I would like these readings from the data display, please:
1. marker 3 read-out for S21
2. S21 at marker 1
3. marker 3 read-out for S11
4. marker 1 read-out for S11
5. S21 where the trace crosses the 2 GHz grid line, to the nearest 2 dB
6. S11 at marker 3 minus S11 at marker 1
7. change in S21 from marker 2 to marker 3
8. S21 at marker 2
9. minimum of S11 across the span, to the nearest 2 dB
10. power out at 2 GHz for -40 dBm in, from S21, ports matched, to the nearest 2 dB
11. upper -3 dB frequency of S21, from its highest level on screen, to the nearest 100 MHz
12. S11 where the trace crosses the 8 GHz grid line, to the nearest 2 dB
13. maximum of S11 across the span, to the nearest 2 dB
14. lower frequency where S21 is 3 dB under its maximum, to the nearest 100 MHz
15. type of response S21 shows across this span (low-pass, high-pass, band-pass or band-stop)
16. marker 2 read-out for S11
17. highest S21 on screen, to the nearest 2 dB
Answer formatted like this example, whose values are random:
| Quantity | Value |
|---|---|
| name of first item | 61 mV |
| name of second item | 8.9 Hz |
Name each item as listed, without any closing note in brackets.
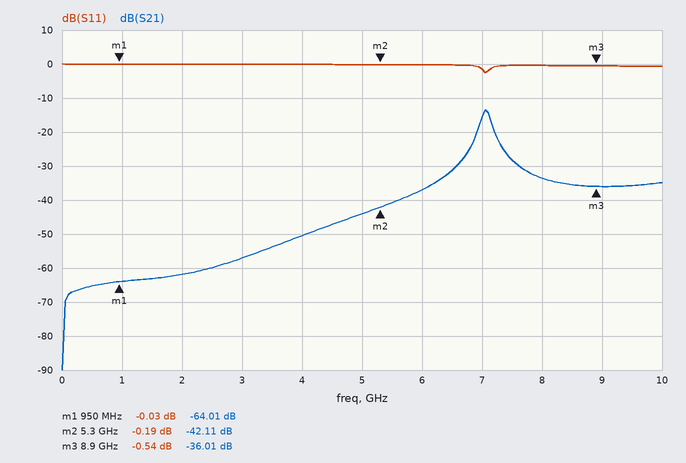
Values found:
| Quantity | Value |
|---|---|
| marker 3 read-out for S21 | -36.01 dB |
| S21 at marker 1 | -64.01 dB |
| marker 3 read-out for S11 | -0.54 dB |
| marker 1 read-out for S11 | -0.03 dB |
| S21 where the trace crosses the 2 GHz grid line, to the nearest 2 dB | -62 dB |
| S11 at marker 3 minus S11 at marker 1 | -0.51 dB |
| change in S21 from marker 2 to marker 3 | 6.10 dB |
| S21 at marker 2 | -42.11 dB |
| minimum of S11 across the span, to the nearest 2 dB | -2 dB |
| power out at 2 GHz for -40 dBm in, from S21, ports matched, to the nearest 2 dB | -102 dBm |
| upper -3 dB frequency of S21, from its highest level on screen, to the nearest 100 MHz | 7.1 GHz |
| S11 where the trace crosses the 8 GHz grid line, to the nearest 2 dB | 0 dB |
| maximum of S11 across the span, to the nearest 2 dB | 0 dB |
| lower frequency where S21 is 3 dB under its maximum, to the nearest 100 MHz | 7.0 GHz |
| type of response S21 shows across this span | band-pass |
| marker 2 read-out for S11 | -0.19 dB |
| highest S21 on screen, to the nearest 2 dB | -14 dB |
